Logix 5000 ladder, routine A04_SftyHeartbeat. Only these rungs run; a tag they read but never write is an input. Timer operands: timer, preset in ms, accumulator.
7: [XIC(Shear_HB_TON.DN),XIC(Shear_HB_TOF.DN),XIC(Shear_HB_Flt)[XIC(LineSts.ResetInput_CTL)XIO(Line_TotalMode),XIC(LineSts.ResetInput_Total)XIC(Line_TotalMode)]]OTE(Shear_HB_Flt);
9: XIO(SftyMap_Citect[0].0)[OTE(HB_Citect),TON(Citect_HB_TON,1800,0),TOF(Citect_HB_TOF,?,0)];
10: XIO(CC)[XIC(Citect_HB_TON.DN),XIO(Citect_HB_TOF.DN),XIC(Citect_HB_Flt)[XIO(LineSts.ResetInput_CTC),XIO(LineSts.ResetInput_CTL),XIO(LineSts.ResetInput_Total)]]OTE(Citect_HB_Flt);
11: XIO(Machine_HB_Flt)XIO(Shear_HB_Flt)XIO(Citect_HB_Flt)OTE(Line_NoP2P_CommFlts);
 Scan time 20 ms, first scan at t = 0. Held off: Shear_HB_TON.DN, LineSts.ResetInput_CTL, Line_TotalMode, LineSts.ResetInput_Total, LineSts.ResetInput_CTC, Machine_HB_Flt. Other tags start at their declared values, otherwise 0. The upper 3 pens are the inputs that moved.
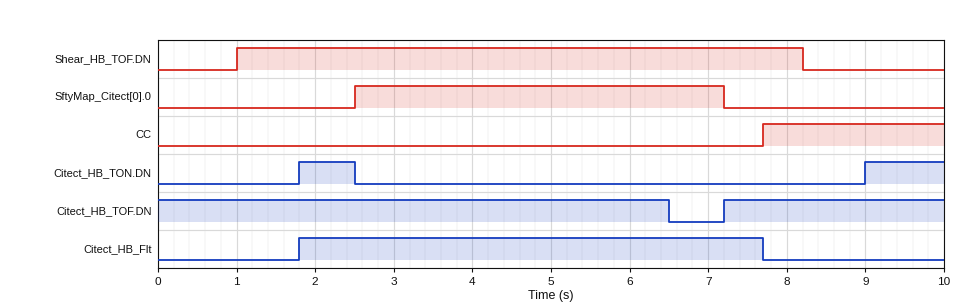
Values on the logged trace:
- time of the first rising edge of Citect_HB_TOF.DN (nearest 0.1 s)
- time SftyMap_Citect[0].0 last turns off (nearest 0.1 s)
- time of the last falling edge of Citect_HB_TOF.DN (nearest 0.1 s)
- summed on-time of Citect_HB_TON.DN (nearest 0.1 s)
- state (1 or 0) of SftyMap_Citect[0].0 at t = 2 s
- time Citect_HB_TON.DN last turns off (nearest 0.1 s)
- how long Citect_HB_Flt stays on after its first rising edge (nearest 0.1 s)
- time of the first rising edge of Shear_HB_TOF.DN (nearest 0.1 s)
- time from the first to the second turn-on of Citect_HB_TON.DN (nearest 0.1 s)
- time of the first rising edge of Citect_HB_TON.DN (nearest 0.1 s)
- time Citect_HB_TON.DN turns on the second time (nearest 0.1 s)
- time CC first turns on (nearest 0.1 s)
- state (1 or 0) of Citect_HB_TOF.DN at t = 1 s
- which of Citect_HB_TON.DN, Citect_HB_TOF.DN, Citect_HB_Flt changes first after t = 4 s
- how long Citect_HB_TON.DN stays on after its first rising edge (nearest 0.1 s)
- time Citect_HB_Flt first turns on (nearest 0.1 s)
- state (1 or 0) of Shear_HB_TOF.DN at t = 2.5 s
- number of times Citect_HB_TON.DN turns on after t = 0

7.2 s
7.2 s
6.5 s
1.7 s
0
2.5 s
5.9 s
1.0 s
7.2 s
1.8 s
9.0 s
7.7 s
1
Citect_HB_TOF.DN
0.7 s
1.8 s
1
2
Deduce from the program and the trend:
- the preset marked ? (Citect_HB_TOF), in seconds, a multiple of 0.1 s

4.0 s
